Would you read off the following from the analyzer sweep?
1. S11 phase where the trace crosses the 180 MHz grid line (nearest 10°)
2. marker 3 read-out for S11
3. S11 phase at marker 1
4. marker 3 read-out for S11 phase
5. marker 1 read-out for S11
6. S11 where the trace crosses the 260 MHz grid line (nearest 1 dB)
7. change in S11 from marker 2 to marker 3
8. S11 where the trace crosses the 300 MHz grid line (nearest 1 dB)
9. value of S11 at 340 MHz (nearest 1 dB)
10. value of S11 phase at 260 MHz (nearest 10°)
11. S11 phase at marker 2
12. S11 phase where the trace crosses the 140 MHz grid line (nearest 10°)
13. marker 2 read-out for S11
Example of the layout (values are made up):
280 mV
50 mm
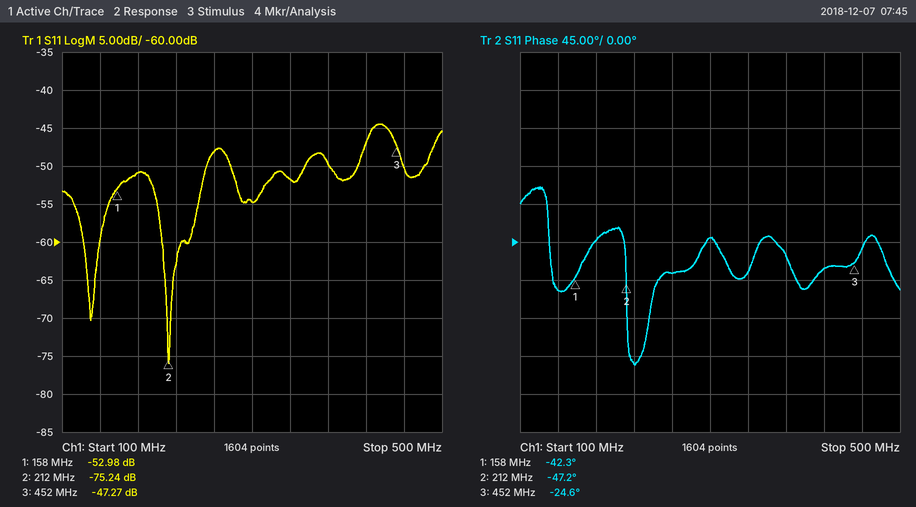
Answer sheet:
0°
-47.27 dB
-42.3°
-24.6°
-52.98 dB
-48 dB
27.97 dB
-55 dB
-52 dB
-40°
-47.2°
-60°
-75.24 dB
